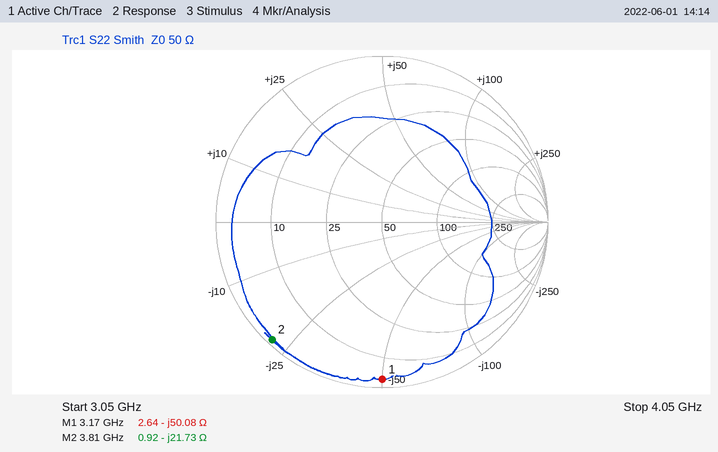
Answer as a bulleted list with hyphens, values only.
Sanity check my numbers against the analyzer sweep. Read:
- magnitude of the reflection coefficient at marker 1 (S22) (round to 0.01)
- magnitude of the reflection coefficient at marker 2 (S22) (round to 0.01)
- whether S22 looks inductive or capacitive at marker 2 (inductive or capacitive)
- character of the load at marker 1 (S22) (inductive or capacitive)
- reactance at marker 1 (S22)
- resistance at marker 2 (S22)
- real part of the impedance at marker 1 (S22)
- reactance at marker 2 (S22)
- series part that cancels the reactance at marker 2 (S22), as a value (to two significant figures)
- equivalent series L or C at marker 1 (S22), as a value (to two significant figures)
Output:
- 0.95
- 0.97
- capacitive
- capacitive
- -50.08 Ω
- 0.92 Ω
- 2.64 Ω
- -21.73 Ω
- 910 pH
- 1.0 pF
